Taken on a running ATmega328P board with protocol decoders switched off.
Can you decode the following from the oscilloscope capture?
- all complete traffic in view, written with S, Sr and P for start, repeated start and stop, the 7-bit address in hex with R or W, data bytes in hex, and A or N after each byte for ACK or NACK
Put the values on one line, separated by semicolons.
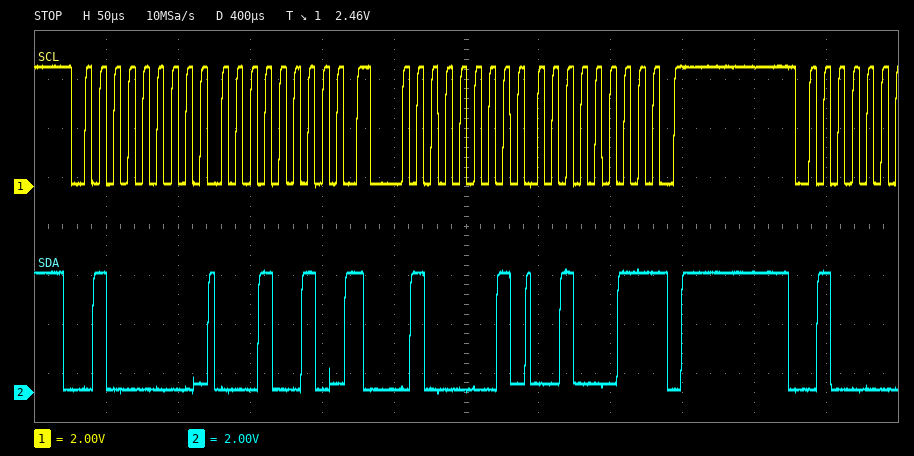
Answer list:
S 20W A 12 A Sr 20R A 23 N P
